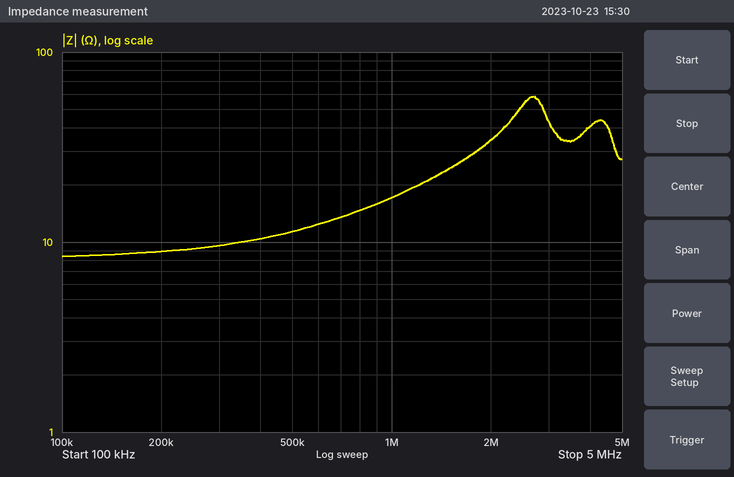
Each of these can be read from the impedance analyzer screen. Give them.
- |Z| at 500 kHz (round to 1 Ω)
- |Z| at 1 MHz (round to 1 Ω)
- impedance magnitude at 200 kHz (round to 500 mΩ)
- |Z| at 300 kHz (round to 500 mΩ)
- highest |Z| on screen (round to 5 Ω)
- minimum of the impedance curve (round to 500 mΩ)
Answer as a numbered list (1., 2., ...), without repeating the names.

1. 11 Ω
2. 17 Ω
3. 9.0 Ω
4. 9.5 Ω
5. 60 Ω
6. 8.5 Ω
